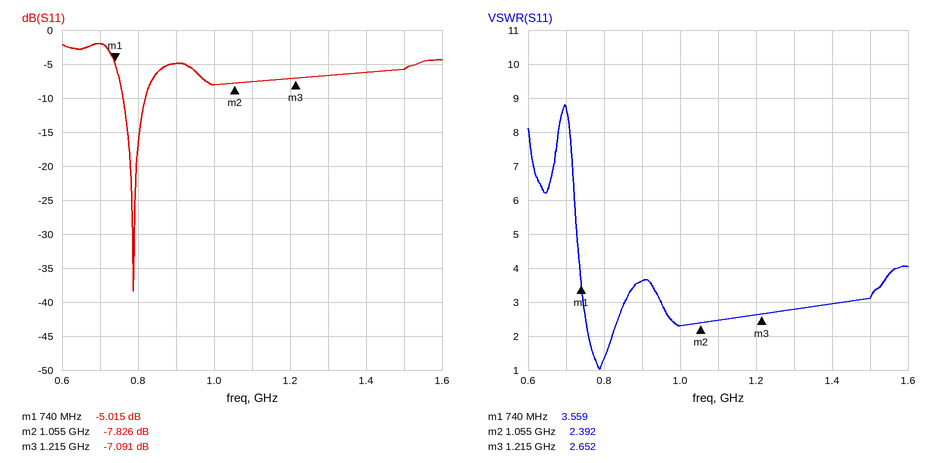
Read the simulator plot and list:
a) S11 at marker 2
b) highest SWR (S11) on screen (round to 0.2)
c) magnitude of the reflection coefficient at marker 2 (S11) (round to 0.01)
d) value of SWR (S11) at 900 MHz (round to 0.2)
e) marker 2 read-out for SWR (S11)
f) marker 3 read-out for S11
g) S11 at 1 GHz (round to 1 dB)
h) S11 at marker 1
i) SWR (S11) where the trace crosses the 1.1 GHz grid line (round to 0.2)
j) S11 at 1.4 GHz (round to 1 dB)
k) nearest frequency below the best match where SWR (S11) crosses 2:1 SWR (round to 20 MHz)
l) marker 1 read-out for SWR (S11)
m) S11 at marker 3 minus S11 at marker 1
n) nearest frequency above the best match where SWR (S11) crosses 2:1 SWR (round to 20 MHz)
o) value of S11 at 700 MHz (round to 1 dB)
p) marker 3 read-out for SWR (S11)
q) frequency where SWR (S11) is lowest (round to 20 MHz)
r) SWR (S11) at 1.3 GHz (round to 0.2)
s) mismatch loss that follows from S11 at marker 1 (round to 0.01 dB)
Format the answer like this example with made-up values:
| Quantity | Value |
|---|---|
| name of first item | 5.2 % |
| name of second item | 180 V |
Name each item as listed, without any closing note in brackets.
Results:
| Quantity | Value |
|---|---|
| S11 at marker 2 | -7.826 dB |
| highest SWR (S11) on screen | 8.8 |
| magnitude of the reflection coefficient at marker 2 (S11) | 0.41 |
| value of SWR (S11) at 900 MHz | 3.6 |
| marker 2 read-out for SWR | 2.392 |
| marker 3 read-out for S11 | -7.091 dB |
| S11 at 1 GHz | -8 dB |
| S11 at marker 1 | -5.015 dB |
| SWR (S11) where the trace crosses the 1.1 GHz grid line | 2.4 |
| S11 at 1.4 GHz | -6 dB |
| nearest frequency below the best match where SWR (S11) crosses 2:1 SWR | 760 MHz |
| marker 1 read-out for SWR | 3.559 |
| S11 at marker 3 minus S11 at marker 1 | -2.076 dB |
| nearest frequency above the best match where SWR (S11) crosses 2:1 SWR | 820 MHz |
| value of S11 at 700 MHz | -2 dB |
| marker 3 read-out for SWR | 2.652 |
| frequency where SWR (S11) is lowest | 780 MHz |
| SWR (S11) at 1.3 GHz | 2.8 |
| mismatch loss that follows from S11 at marker 1 | 1.64 dB |
